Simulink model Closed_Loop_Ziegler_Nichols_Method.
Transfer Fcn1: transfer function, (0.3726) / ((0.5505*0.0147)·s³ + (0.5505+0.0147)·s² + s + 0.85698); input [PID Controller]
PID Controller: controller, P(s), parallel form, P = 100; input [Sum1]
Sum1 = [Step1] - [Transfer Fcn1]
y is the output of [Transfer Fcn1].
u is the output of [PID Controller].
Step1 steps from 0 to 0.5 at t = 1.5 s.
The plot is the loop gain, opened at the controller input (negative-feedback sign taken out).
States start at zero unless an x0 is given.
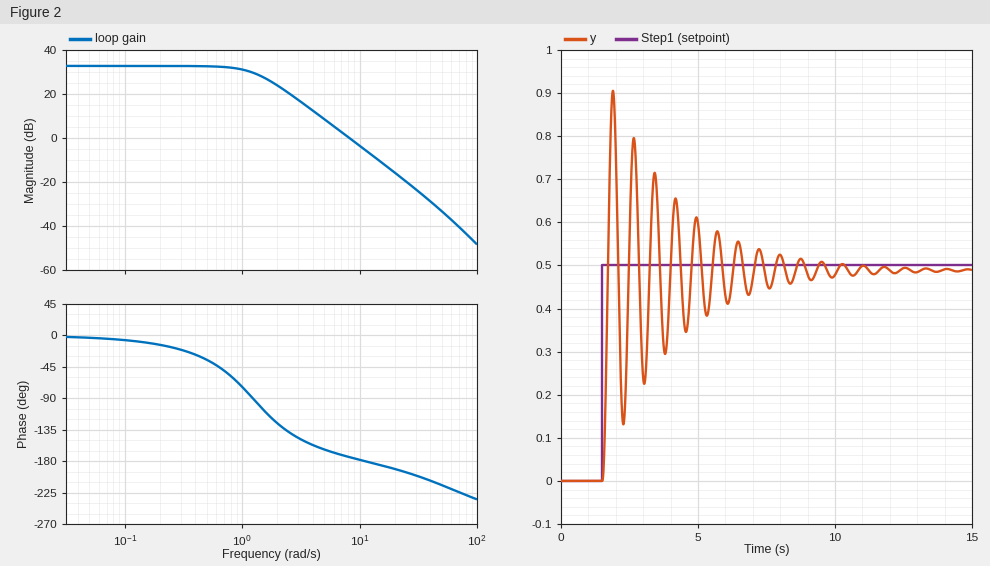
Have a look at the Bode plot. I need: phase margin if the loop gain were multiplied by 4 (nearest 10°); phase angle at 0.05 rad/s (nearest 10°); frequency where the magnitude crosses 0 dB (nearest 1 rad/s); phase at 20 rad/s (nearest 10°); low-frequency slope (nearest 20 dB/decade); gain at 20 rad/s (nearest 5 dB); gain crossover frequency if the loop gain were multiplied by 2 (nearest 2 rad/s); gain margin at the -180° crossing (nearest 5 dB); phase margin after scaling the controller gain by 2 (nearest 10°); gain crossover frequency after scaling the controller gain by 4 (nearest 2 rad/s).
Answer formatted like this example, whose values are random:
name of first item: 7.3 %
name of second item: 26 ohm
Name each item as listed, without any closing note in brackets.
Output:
phase margin if the loop gain were multiplied by 4: -10°
phase angle at 0.05 rad/s: 0°
frequency where the magnitude crosses 0 dB: 8 rad/s
phase at 20 rad/s: -190°
low-frequency slope: 0 dB/decade
gain at 20 rad/s: -15 dB
gain crossover frequency if the loop gain were multiplied by 2: 12 rad/s
gain margin at the -180° crossing: 5 dB
phase margin after scaling the controller gain by 2: 0°
gain crossover frequency after scaling the controller gain by 4: 16 rad/s
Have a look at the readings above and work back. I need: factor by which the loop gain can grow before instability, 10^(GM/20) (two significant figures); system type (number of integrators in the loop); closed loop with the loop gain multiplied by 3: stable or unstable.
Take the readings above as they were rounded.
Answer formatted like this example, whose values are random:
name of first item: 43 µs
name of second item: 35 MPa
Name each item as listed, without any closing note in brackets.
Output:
factor by which the loop gain can grow before instability, 10^(GM/20): 1.8
system type: 0
closed loop with the loop gain multiplied by 3: stable or unstable: unstable
